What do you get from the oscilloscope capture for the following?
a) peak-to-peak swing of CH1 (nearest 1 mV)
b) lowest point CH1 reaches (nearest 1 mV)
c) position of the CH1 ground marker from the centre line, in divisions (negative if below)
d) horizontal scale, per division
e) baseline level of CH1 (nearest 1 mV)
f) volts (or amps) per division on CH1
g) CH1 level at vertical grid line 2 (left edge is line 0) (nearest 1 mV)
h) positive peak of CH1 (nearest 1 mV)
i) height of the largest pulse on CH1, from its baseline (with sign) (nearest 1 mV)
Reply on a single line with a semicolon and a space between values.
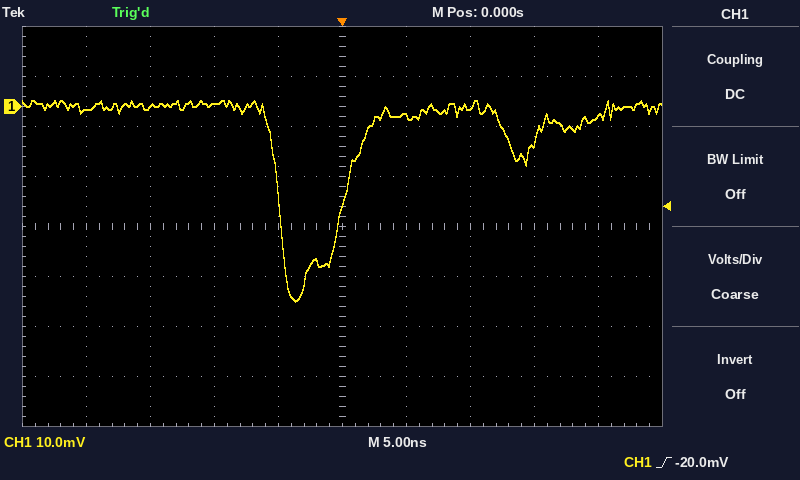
40 mV; -39 mV; +2.4 div; 5 ns; 0 mV; 10 mV; 0 mV; 1 mV; -39 mV
